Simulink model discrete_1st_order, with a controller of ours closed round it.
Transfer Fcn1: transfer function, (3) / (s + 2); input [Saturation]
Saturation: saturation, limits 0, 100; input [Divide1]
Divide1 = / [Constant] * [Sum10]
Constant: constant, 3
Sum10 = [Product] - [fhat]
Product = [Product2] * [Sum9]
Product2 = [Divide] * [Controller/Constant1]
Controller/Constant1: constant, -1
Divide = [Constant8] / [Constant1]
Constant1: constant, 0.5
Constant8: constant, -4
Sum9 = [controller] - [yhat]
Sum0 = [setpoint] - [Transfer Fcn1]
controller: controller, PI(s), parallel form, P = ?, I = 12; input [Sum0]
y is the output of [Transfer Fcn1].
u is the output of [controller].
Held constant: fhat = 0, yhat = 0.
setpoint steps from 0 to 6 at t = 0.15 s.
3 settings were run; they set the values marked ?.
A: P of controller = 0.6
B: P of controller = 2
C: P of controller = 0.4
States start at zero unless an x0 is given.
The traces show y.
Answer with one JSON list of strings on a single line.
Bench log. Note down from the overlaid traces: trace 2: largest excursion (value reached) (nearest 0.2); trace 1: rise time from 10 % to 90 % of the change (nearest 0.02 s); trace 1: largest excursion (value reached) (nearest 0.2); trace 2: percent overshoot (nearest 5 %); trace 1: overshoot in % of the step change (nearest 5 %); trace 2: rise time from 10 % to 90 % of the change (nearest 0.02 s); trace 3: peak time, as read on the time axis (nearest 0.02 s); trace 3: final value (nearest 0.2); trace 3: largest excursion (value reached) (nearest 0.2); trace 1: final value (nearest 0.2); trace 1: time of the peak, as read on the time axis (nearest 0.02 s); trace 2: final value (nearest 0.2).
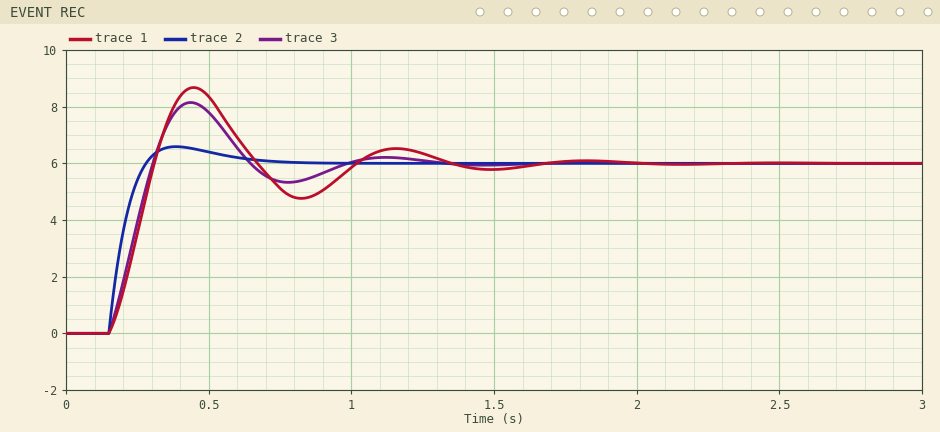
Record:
["6.6", "0.12 s", "8.6", "10 %", "45 %", "0.10 s", "0.44 s", "6.0", "8.2", "6.0", "0.44 s", "6.0"]
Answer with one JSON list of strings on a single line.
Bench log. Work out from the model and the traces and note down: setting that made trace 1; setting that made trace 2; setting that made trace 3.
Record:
["C", "B", "A"]
